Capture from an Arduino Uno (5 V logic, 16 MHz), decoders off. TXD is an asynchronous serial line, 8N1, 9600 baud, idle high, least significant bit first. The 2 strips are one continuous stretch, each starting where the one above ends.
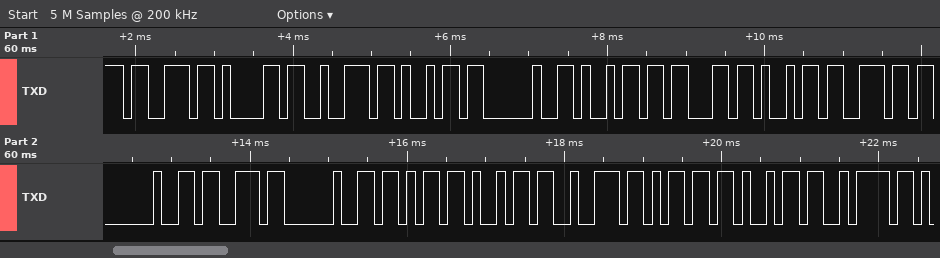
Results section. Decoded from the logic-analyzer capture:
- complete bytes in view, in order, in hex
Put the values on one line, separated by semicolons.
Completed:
0x73 0x61 0x72 0x69 0x20 0x69 0x63 0x69 0x6E 0x20 0x73 0x20 0x6B 0x69 0x72 0x6D 0x69 0x7A
